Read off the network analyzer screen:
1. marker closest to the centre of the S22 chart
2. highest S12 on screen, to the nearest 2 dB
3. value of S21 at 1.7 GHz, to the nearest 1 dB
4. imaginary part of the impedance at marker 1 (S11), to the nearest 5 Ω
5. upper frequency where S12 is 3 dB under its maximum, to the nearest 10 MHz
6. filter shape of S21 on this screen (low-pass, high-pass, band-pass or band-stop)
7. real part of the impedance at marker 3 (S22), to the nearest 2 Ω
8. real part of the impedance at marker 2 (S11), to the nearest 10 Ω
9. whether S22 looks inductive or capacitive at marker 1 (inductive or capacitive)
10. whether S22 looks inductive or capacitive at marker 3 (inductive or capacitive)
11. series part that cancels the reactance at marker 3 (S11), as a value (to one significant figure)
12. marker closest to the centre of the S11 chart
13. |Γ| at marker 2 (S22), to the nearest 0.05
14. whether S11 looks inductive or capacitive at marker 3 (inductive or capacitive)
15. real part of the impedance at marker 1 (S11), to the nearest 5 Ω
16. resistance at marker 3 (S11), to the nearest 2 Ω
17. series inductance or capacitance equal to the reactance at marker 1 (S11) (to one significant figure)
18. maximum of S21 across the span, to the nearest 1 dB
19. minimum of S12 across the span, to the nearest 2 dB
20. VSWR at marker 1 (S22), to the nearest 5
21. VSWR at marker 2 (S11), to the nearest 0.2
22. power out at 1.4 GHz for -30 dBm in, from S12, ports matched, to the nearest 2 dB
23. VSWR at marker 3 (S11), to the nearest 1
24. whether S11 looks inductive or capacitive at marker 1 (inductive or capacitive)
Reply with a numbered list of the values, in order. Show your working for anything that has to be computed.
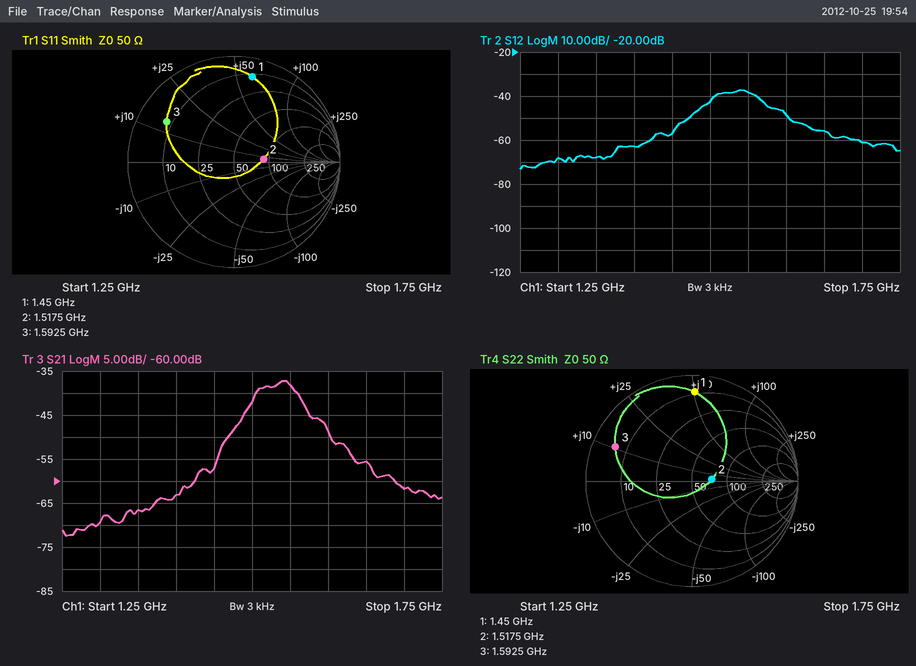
1. marker 2
2. -38 dB
3. -62 dB
4. +60 Ω
5. 1.56 GHz
6. band-pass
7. 6 Ω
8. 90 Ω
9. inductive
10. inductive
11. C = 1/(2π × 1.5925 GHz × 14 Ω) ≈ 7 pF
12. marker 2
13. 0.20
14. inductive
15. 10 Ω
16. 8 Ω
17. L = 60 Ω/(2π × 1.45 GHz) ≈ 7 nH
18. -37 dB
19. -74 dB
20. 10
21. 1.8
22. -30 dBm + (-62 dB) = -92 dBm
23. 7
24. inductive
